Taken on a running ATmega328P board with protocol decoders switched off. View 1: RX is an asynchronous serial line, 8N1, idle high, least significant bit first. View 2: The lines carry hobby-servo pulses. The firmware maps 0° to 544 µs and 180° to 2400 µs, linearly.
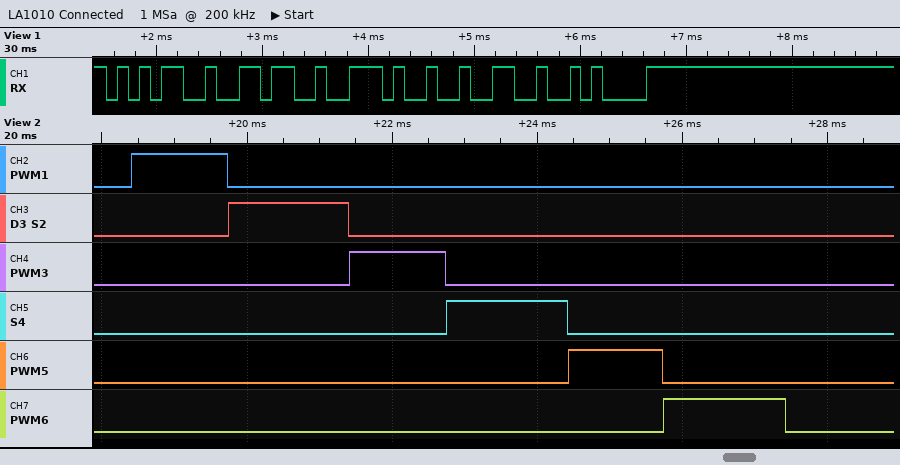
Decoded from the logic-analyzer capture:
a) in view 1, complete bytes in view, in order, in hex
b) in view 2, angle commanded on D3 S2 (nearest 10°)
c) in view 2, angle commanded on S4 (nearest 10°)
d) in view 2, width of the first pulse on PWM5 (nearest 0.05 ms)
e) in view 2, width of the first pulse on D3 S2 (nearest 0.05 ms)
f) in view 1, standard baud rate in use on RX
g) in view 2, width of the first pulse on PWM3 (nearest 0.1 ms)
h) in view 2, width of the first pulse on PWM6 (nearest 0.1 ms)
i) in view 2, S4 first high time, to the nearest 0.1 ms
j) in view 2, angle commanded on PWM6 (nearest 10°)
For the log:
0x35 0x36 0x2E 0x32 0x0A
110°
110°
1.30 ms
1.65 ms
9600 baud
1.3 ms
1.7 ms
1.7 ms
110°
